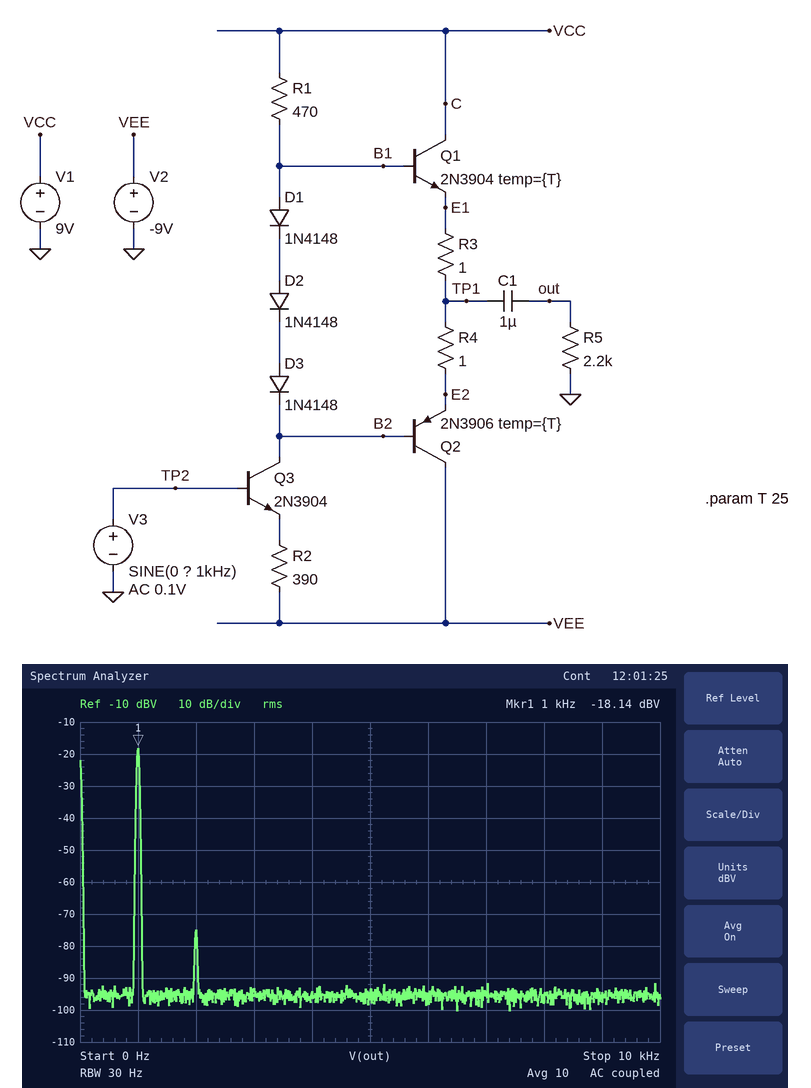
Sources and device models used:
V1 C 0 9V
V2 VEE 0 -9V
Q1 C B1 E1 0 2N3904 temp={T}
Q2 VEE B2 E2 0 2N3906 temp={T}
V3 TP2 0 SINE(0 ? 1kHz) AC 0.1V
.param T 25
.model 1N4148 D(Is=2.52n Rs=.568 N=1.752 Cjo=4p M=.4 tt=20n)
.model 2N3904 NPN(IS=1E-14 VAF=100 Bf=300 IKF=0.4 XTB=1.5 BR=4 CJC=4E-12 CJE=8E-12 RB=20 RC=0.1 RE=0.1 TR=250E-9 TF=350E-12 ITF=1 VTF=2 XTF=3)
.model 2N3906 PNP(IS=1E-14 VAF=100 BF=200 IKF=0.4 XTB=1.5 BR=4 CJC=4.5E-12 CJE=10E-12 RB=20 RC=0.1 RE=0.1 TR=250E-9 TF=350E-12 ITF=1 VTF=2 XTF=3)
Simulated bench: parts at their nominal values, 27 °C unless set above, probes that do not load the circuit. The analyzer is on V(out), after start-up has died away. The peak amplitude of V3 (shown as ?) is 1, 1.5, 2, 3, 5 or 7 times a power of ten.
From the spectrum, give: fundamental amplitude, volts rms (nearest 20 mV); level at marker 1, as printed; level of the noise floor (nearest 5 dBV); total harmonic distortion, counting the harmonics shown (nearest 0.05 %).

120 mV
-18.14 dBV
-95 dBV
0.15 %
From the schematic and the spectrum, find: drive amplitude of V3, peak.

200 mV
